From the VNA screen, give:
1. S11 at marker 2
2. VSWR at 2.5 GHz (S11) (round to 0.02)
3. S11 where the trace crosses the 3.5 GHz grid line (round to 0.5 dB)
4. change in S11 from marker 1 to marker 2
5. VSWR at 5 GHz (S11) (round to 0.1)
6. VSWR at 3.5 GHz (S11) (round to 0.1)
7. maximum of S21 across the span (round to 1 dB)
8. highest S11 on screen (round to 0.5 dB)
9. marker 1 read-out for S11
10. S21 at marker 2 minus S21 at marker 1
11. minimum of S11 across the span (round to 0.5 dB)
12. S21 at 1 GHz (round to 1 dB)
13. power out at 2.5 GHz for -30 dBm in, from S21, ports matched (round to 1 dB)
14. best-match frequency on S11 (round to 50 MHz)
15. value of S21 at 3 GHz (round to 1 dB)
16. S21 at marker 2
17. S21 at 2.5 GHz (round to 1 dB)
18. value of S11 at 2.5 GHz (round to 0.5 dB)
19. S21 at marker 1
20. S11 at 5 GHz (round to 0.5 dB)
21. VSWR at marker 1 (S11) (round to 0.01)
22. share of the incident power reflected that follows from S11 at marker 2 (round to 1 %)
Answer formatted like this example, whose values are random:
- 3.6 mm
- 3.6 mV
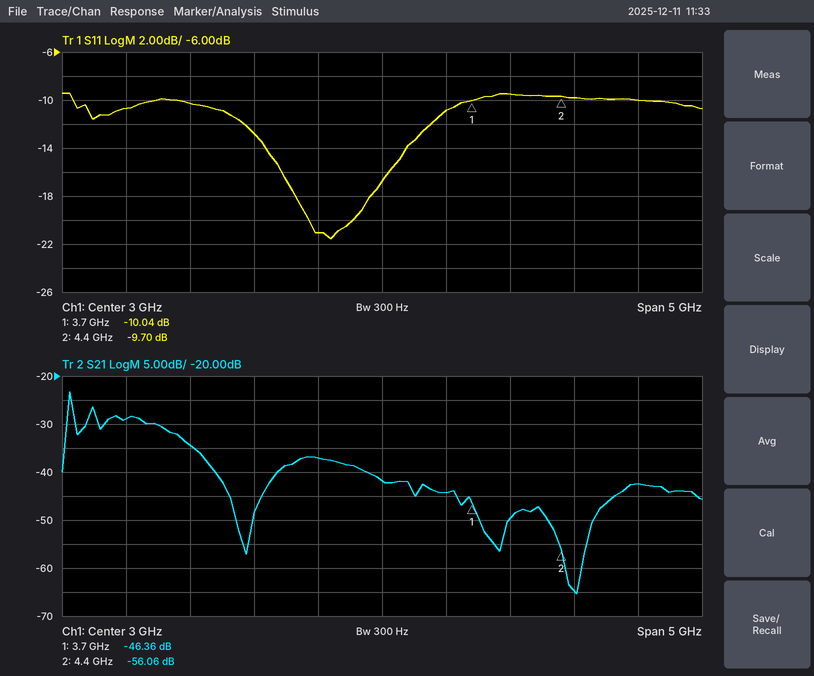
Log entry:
- -9.70 dB
- 1.20
- -11.0 dB
- 0.34 dB
- 1.9
- 1.8
- -23 dB
- -9.5 dB
- -10.04 dB
- -9.70 dB
- -21.5 dB
- -29 dB
- -67 dBm
- 2.60 GHz
- -42 dB
- -56.06 dB
- -37 dB
- -21.0 dB
- -46.36 dB
- -10.0 dB
- 1.92
- 11 %
